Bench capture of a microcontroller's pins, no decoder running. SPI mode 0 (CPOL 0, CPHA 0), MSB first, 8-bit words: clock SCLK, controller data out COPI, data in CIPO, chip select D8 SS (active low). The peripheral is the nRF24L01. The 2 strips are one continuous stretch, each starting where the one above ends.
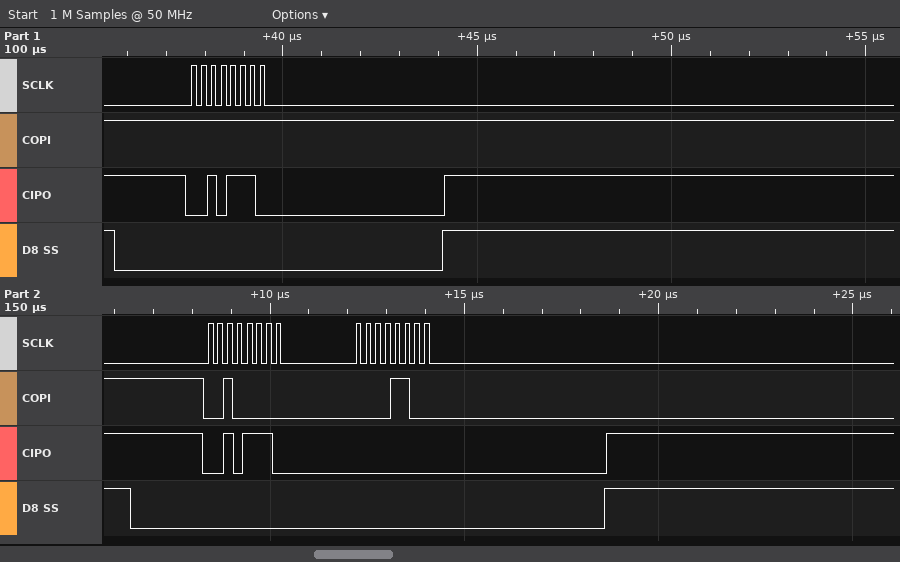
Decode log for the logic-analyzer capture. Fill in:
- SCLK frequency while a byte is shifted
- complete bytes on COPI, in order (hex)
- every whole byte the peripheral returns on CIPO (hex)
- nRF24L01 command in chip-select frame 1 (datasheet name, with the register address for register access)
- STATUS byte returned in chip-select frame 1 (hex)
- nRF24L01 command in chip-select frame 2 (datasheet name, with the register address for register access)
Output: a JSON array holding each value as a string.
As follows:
["4 MHz", "FF 20 0C", "2E 2E 00", "NOP", "0x2E", "W_REGISTER 0x00"]
